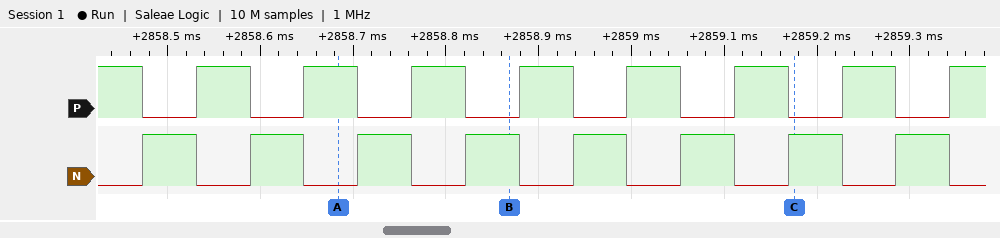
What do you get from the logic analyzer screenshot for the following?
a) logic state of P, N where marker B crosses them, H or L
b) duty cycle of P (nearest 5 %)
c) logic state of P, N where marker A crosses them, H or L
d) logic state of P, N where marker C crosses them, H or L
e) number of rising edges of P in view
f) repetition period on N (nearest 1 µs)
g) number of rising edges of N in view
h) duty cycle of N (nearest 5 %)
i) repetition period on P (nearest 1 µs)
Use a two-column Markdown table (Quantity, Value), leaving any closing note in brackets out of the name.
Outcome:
| Quantity | Value |
|---|---|
| logic state of P, N where marker B crosses them, H or L | P=L, N=H |
| duty cycle of P | 50 % |
| logic state of P, N where marker A crosses them, H or L | P=H, N=L |
| logic state of P, N where marker C crosses them, H or L | P=L, N=H |
| number of rising edges of P in view | 8 |
| repetition period on N | 116 µs |
| number of rising edges of N in view | 8 |
| duty cycle of N | 50 % |
| repetition period on P | 116 µs |
